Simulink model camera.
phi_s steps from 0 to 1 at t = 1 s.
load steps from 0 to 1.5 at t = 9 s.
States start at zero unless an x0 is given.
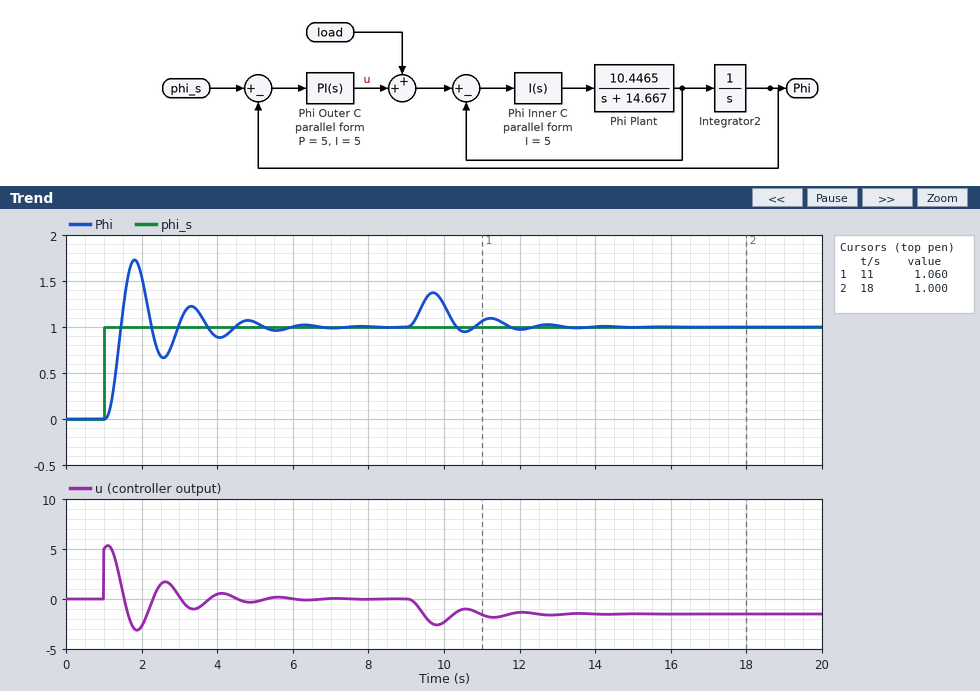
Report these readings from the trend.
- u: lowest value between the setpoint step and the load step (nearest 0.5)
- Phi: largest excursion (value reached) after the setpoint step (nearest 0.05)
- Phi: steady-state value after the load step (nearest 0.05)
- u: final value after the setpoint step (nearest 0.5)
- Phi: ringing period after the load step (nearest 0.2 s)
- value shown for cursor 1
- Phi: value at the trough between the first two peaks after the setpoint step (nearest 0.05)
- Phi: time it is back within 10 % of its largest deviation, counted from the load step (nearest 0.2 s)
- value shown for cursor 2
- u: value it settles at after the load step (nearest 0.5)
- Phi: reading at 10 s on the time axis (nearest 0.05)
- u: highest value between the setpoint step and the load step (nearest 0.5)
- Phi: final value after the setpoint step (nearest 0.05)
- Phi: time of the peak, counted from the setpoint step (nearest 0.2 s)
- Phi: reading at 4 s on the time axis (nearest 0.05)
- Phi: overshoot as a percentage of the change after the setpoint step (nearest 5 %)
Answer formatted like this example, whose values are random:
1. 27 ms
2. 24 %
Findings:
1. -3.0
2. 1.75
3. 1.00
4. 0.0
5. 1.6 s
6. 1.060
7. 0.65
8. 2.6 s
9. 1.000
10. -1.5
11. 1.25
12. 5.5
13. 1.00
14. 0.8 s
15. 0.90
16. 75 %
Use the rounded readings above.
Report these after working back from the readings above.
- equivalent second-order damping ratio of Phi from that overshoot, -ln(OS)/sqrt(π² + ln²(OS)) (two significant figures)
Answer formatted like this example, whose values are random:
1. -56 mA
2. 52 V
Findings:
1. 0.091
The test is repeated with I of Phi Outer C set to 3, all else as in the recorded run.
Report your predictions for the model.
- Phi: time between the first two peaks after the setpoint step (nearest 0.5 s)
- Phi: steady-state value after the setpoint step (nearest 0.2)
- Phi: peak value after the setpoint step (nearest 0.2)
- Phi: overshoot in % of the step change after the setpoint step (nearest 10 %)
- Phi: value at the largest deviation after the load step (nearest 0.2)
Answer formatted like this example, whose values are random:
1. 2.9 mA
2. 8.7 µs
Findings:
1. 1.5 s
2. 1.0
3. 1.6
4. 60 %
5. 1.4
